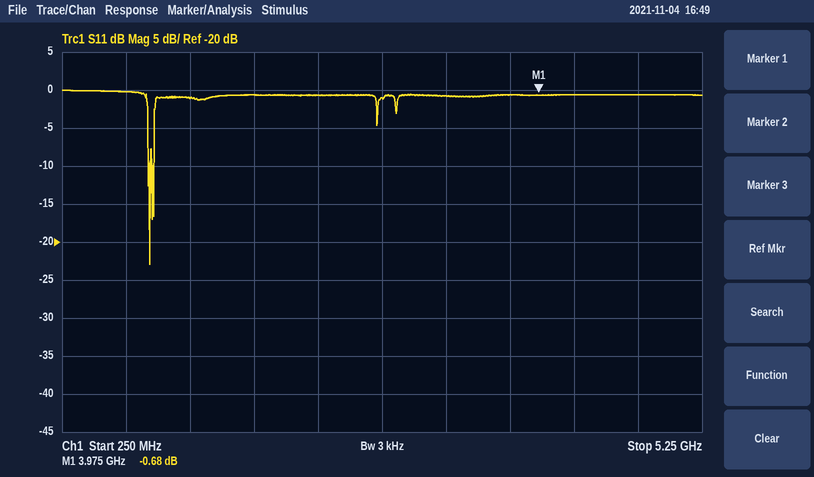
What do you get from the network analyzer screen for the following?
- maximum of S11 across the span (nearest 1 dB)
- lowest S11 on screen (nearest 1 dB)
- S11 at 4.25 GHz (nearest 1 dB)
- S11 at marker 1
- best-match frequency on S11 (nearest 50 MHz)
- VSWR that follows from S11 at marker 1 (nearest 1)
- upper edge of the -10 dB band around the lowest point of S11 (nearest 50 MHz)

0 dB
-23 dB
-1 dB
-0.68 dB
950 MHz
26
950 MHz
